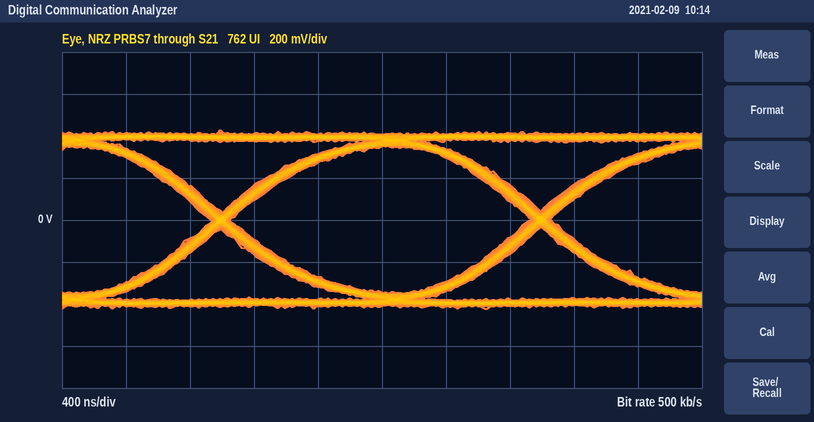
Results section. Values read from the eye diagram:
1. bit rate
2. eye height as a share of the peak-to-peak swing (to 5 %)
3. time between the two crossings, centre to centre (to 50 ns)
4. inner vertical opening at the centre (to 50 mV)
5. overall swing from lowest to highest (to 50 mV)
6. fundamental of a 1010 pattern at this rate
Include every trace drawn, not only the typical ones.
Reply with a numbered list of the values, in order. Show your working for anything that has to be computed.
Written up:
1. 500 kb/s
2. 700 mV / 850 mV ≈ 82.4 %, so 80 % to the nearest 5 %
3. 2.00 µs
4. 700 mV
5. 850 mV
6. 250 kHz
